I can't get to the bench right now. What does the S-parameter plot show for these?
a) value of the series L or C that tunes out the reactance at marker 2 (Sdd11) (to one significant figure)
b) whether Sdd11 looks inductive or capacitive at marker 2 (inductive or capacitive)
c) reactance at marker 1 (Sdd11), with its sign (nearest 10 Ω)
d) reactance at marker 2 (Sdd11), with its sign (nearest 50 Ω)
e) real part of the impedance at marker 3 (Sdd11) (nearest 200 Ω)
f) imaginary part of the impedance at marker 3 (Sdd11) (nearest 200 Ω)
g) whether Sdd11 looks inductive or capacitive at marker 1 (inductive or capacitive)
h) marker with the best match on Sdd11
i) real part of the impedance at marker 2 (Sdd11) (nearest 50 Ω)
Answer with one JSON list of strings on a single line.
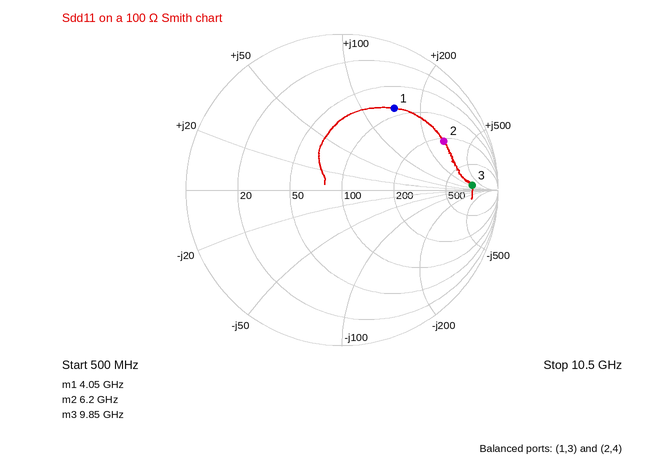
["90 fF", "inductive", "+150 Ω", "+300 Ω", "1000 Ω", "+200 Ω", "inductive", "marker 1", "200 Ω"]
